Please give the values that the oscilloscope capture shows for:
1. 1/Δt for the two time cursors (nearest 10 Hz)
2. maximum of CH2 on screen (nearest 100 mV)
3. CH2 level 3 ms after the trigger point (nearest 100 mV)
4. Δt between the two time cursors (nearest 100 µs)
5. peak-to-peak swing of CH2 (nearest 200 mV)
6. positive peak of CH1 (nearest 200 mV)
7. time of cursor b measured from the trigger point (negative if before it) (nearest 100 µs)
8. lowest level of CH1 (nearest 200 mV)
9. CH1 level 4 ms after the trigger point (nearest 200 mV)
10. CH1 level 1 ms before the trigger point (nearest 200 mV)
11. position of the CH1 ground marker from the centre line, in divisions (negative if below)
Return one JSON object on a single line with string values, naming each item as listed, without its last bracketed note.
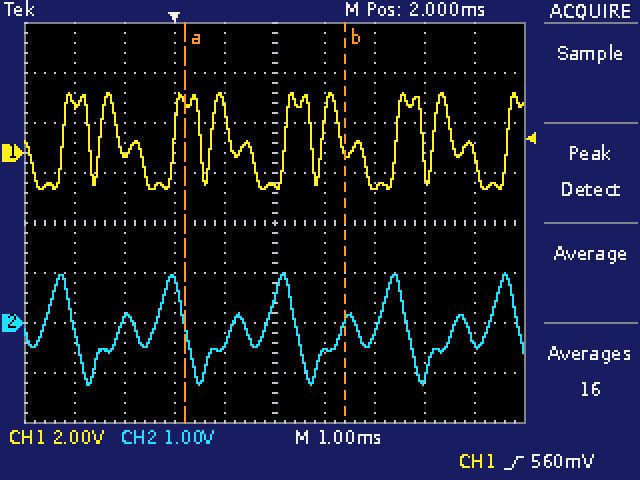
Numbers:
{"1/Δt for the two time cursors": "310 Hz", "maximum of CH2 on screen": "1.0 V", "CH2 level 3 ms after the trigger point": "-600 mV", "Δt between the two time cursors": "3.2 ms", "peak-to-peak swing of CH2": "2.2 V", "positive peak of CH1": "2.4 V", "time of cursor b measured from the trigger point (negative if before it)": "+3.4 ms", "lowest level of CH1": "-1.4 V", "CH1 level 4 ms after the trigger point": "-1.4 V", "CH1 level 1 ms before the trigger point": "0.0 V", "position of the CH1 ground marker from the centre line, in divisions": "+1.4 div"}
